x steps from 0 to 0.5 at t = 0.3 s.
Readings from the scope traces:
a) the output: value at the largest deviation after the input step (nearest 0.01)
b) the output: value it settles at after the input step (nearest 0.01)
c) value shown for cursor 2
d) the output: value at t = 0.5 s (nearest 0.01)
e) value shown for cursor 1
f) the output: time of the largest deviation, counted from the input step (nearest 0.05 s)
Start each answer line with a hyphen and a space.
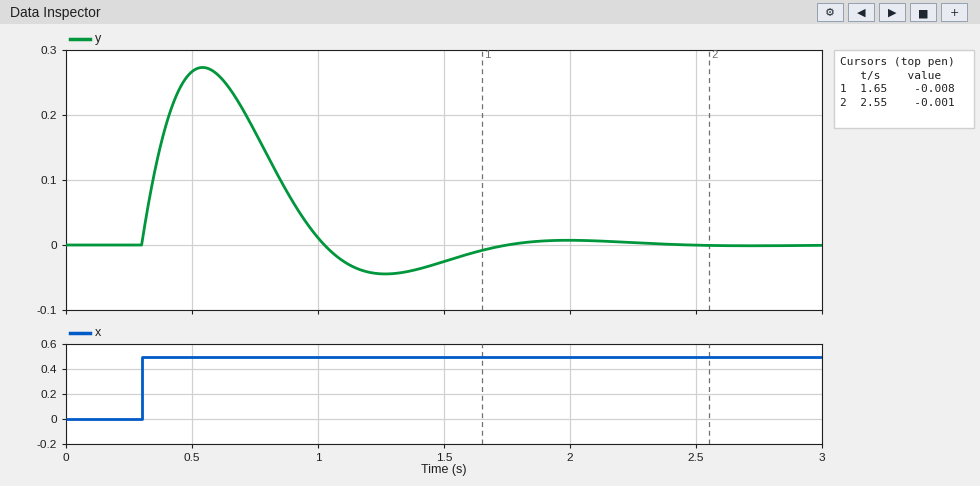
- 0.27
- 0.00
- -0.001
- 0.27
- -0.008
- 0.25 s
